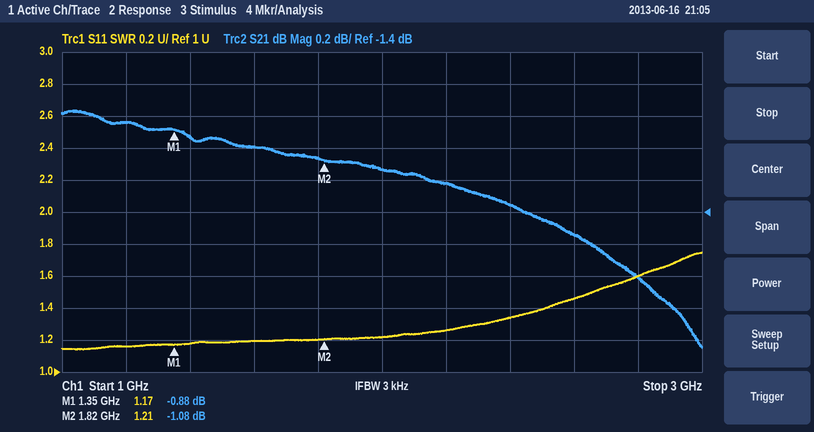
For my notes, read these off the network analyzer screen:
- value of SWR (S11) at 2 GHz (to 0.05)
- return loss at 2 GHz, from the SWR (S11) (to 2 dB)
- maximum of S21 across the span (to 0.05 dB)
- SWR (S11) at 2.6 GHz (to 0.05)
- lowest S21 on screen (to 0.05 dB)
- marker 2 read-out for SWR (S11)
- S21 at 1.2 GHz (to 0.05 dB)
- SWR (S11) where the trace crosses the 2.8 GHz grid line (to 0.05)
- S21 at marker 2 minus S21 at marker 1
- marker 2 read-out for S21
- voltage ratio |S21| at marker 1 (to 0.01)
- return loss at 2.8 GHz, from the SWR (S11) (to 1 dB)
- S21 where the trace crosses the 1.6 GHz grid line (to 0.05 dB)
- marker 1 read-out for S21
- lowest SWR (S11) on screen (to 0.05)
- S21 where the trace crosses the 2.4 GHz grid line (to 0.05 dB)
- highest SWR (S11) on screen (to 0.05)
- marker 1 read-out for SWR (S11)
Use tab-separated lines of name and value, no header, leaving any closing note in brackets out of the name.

value of SWR (S11) at 2 GHz	1.20
return loss at 2 GHz, from the SWR (S11)	20 dB
maximum of S21 across the span	-0.75 dB
SWR (S11) at 2.6 GHz	1.45
lowest S21 on screen	-2.25 dB
marker 2 read-out for SWR	1.21
S21 at 1.2 GHz	-0.85 dB
SWR (S11) where the trace crosses the 2.8 GHz grid line	1.60
S21 at marker 2 minus S21 at marker 1	-0.20 dB
marker 2 read-out for S21	-1.08 dB
voltage ratio |S21| at marker 1	0.90
return loss at 2.8 GHz, from the SWR (S11)	13 dB
S21 where the trace crosses the 1.6 GHz grid line	-1.00 dB
marker 1 read-out for S21	-0.88 dB
lowest SWR (S11) on screen	1.15
S21 where the trace crosses the 2.4 GHz grid line	-1.35 dB
highest SWR (S11) on screen	1.75
marker 1 read-out for SWR	1.17
